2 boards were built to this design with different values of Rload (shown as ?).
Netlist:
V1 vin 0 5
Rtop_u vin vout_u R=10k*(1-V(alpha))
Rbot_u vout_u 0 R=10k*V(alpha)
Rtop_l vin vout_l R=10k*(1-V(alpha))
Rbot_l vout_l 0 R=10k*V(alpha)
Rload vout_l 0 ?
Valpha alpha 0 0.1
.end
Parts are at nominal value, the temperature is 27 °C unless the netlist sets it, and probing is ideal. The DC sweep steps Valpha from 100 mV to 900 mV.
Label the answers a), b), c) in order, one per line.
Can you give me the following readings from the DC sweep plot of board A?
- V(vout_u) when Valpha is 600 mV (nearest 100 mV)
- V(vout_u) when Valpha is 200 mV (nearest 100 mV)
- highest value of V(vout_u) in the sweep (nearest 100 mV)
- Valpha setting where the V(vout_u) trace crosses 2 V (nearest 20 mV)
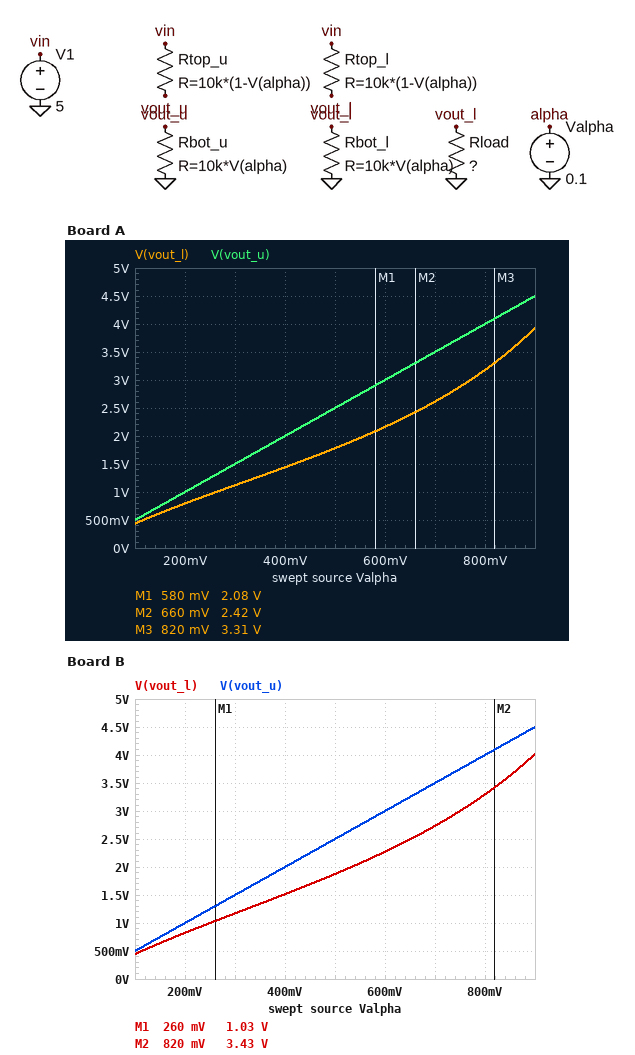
a) 3.0 V
b) 1.0 V
c) 4.5 V
d) 400 mV
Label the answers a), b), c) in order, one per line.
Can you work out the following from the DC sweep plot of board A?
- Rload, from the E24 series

a) 6.2 kΩ
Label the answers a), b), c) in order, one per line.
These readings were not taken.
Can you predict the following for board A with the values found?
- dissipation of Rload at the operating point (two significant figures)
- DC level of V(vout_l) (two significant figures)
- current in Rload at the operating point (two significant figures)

a) 31 µW
b) 440 mV
c) 70 µA
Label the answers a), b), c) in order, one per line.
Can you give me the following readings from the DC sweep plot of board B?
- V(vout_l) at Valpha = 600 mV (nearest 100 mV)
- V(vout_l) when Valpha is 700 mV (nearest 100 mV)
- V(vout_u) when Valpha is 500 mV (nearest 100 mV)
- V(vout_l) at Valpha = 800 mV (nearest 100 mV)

a) 2.3 V
b) 2.7 V
c) 2.5 V
d) 3.3 V
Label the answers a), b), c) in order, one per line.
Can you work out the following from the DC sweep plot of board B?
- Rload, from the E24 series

a) 7.5 kΩ
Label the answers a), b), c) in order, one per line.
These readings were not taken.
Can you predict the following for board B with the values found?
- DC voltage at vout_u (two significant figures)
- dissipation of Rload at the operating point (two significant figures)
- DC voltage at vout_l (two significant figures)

a) 500 mV
b) 27 µW
c) 450 mV
